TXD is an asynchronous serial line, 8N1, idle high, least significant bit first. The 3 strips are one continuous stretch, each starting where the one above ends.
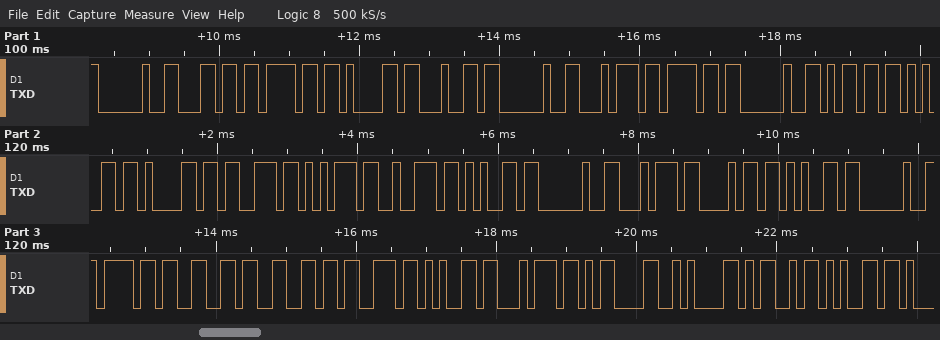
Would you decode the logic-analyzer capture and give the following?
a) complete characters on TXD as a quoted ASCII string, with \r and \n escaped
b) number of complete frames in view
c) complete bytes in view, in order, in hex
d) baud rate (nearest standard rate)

" load to measure the offset\r\nMe"
31
20 6C 6F 61 64 20 74 6F 20 6D 65 61 73 75 72 65 20 74 68 65 20 6F 66 66 73 65 74 0D 0A 4D 65
9600 baud
